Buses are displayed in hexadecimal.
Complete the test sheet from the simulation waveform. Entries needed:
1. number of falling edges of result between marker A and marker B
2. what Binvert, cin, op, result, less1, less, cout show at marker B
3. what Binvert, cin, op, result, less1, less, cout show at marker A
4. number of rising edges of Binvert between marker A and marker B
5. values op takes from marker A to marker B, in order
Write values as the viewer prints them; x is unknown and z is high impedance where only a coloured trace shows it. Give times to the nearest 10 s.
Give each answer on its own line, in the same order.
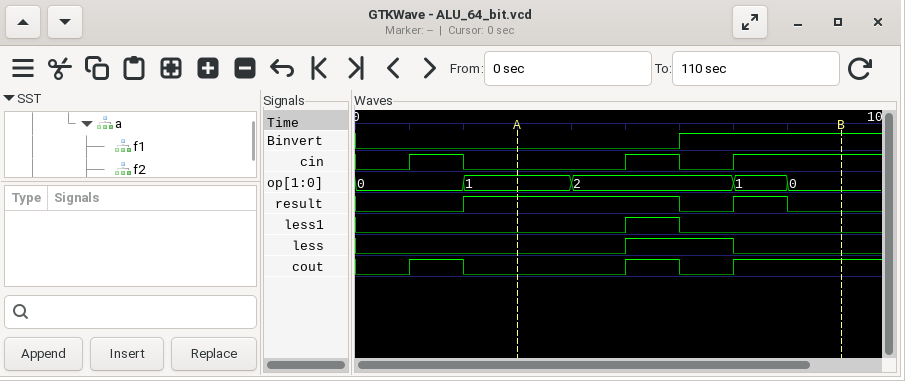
2
Binvert=1, cin=1, op=0, result=0, less1=0, less=0, cout=1
Binvert=0, cin=0, op=1, result=1, less1=0, less=0, cout=0
1
1, 2, 1, 0
